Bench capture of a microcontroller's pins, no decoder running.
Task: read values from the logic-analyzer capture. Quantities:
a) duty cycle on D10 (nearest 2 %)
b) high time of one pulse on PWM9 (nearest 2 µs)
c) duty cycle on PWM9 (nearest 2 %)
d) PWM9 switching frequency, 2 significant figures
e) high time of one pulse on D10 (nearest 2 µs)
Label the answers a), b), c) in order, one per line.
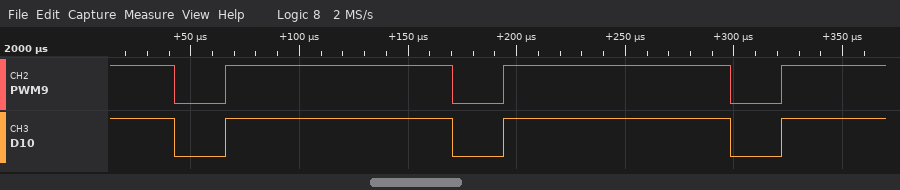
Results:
a) 82 %
b) 104 µs
c) 82 %
d) 7.8 kHz
e) 104 µs
